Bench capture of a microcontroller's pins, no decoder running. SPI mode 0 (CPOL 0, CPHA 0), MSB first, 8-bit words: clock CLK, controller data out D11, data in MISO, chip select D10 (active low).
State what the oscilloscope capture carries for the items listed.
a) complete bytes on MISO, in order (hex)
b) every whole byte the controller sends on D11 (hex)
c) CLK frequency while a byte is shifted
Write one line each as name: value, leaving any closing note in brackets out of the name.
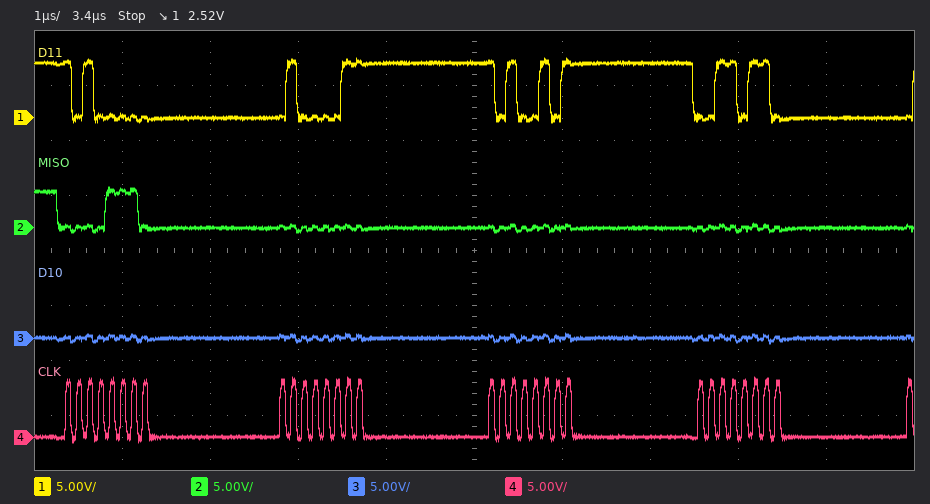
complete bytes on MISO, in order: 0E 00 00 00
every whole byte the controller sends on D11: A0 43 A5 36
CLK frequency while a byte is shifted: 8 MHz
